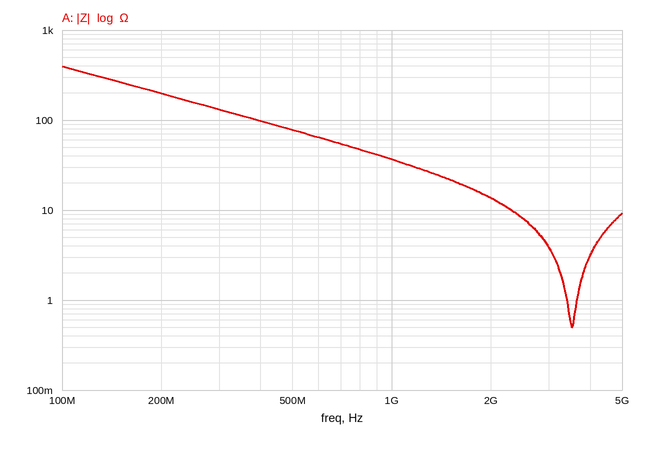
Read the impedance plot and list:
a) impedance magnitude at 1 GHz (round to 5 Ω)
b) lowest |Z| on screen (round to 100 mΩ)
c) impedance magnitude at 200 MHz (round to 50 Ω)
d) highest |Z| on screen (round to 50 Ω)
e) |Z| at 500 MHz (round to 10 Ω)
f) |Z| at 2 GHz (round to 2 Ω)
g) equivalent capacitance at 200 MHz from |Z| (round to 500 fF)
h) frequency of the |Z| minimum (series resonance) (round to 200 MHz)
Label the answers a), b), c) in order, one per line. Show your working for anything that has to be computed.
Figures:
a) 35 Ω
b) 500 mΩ
c) 200 Ω
d) 400 Ω
e) 80 Ω
f) 14 Ω
g) C = 1/(2π × 200 MHz × 200 Ω) ≈ 4.0 pF
h) 3.6 GHz
